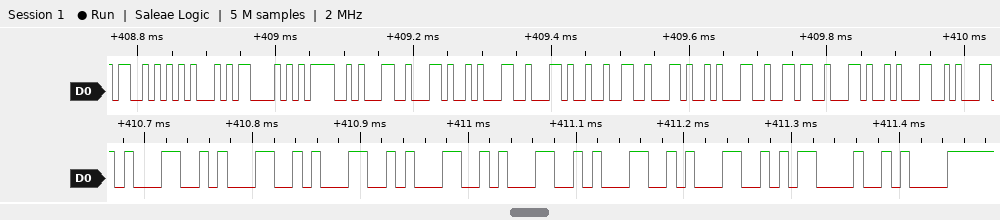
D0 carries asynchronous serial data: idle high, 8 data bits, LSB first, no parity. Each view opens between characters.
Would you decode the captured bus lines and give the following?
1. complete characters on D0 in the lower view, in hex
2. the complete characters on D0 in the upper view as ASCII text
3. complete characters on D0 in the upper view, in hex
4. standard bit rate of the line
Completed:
31, 31, 31, 31, 31, 31, 31, 0D, 0A
"SEC=1,1,2,16,1"
53, 45, 43, 3D, 31, 2C, 31, 2C, 32, 2C, 31, 36, 2C, 31
115200 baud
